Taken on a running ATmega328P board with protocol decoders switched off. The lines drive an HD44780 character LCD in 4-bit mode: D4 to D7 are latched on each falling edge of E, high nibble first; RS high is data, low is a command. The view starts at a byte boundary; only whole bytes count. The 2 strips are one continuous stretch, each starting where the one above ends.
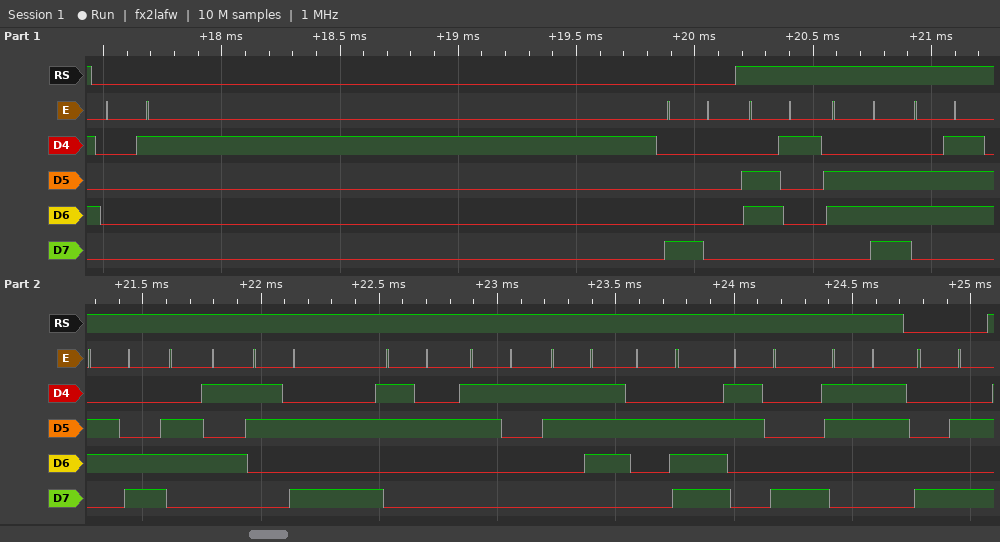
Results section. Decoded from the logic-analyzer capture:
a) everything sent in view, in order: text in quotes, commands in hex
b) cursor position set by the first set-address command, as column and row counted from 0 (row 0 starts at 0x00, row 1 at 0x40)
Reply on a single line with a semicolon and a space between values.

0x01 0x80 "angle:217.83" 0x8A; column 0, row 0
